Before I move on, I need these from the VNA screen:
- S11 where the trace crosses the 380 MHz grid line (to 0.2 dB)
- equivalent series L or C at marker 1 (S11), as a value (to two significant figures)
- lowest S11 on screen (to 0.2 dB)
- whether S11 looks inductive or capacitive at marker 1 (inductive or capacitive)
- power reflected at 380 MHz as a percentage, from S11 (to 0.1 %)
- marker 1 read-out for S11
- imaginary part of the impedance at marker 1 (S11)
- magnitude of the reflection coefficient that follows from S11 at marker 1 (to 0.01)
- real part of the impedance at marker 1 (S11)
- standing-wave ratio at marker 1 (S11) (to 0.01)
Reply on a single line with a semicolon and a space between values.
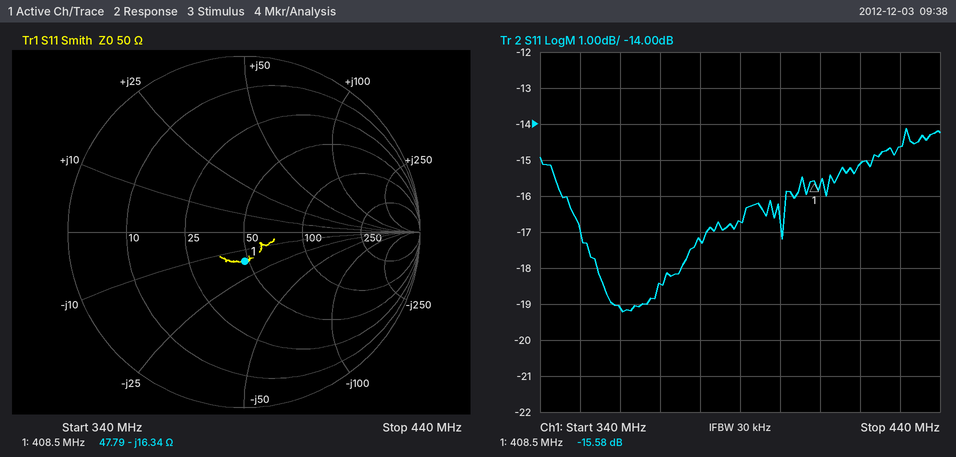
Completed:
-17.2 dB; 24 pF; -19.2 dB; capacitive; 1.9 %; -15.58 dB; -16.34 Ω; 0.17; 47.79 Ω; 1.40
